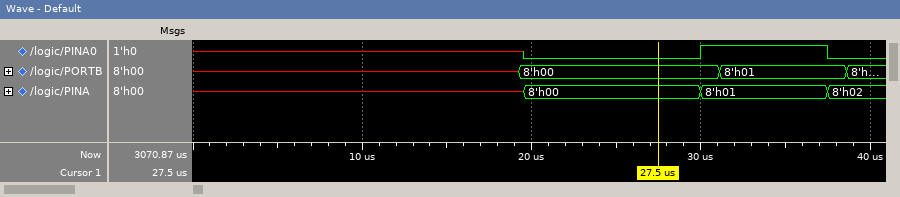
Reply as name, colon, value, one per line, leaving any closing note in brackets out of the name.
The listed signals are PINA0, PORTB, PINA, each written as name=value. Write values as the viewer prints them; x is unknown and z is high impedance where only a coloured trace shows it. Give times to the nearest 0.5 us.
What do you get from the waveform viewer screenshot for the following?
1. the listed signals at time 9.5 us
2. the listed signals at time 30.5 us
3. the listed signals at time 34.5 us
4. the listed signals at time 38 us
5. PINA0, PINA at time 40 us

the listed signals at time 9.5 us: PINA0=x, PORTB=x, PINA=x
the listed signals at time 30.5 us: PINA0=1, PORTB=8'h00, PINA=8'h01
the listed signals at time 34.5 us: PINA0=1, PORTB=8'h01, PINA=8'h01
the listed signals at time 38 us: PINA0=0, PORTB=8'h01, PINA=8'h02
PINA0, PINA at time 40 us: PINA0=0, PINA=8'h02
